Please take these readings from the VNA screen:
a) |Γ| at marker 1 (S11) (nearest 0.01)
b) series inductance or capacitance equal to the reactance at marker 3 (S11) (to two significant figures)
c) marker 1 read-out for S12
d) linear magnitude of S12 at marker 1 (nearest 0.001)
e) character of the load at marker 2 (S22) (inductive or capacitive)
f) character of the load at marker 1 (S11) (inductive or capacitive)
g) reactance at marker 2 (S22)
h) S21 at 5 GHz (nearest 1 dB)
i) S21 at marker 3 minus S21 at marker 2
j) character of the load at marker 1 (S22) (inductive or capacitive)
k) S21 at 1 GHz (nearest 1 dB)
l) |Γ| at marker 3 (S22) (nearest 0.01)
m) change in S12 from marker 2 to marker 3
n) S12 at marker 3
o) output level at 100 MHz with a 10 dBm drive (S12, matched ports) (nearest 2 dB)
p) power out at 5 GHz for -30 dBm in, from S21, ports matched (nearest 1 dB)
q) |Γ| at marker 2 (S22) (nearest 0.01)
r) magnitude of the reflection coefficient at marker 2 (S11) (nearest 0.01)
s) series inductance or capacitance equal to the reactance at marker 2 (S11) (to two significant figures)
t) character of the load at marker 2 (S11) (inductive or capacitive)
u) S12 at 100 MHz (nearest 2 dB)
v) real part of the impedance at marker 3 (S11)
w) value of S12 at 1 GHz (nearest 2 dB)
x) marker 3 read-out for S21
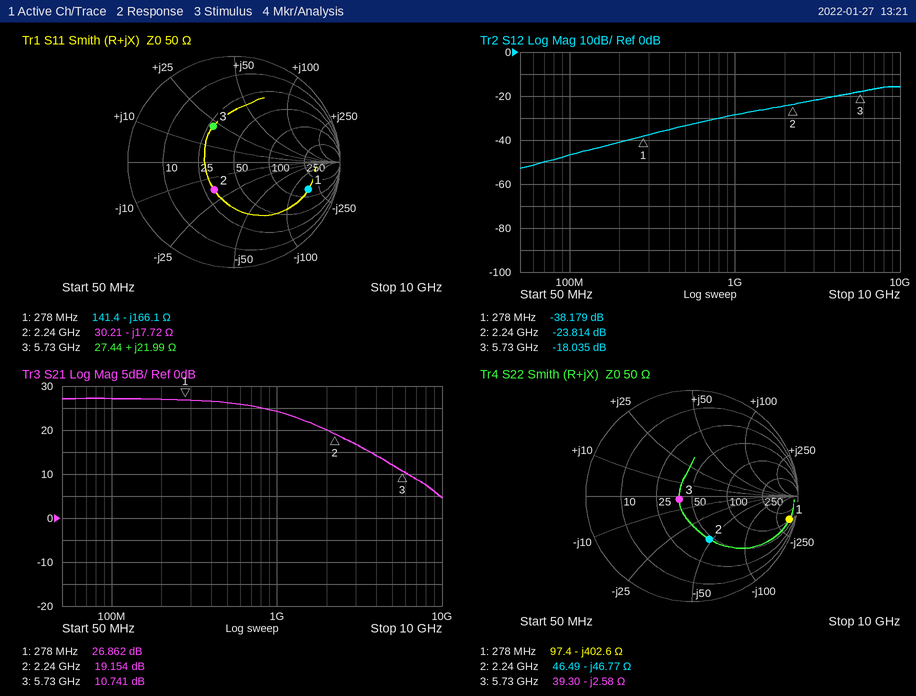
0.75
610 pH
-38.179 dB
0.012
capacitive
capacitive
-46.77 Ω
12 dB
-8.413 dB
capacitive
24 dB
0.12
5.779 dB
-18.035 dB
-36 dBm
-18 dBm
0.44
0.32
4.0 pF
capacitive
-46 dB
27.44 Ω
-28 dB
10.741 dB
